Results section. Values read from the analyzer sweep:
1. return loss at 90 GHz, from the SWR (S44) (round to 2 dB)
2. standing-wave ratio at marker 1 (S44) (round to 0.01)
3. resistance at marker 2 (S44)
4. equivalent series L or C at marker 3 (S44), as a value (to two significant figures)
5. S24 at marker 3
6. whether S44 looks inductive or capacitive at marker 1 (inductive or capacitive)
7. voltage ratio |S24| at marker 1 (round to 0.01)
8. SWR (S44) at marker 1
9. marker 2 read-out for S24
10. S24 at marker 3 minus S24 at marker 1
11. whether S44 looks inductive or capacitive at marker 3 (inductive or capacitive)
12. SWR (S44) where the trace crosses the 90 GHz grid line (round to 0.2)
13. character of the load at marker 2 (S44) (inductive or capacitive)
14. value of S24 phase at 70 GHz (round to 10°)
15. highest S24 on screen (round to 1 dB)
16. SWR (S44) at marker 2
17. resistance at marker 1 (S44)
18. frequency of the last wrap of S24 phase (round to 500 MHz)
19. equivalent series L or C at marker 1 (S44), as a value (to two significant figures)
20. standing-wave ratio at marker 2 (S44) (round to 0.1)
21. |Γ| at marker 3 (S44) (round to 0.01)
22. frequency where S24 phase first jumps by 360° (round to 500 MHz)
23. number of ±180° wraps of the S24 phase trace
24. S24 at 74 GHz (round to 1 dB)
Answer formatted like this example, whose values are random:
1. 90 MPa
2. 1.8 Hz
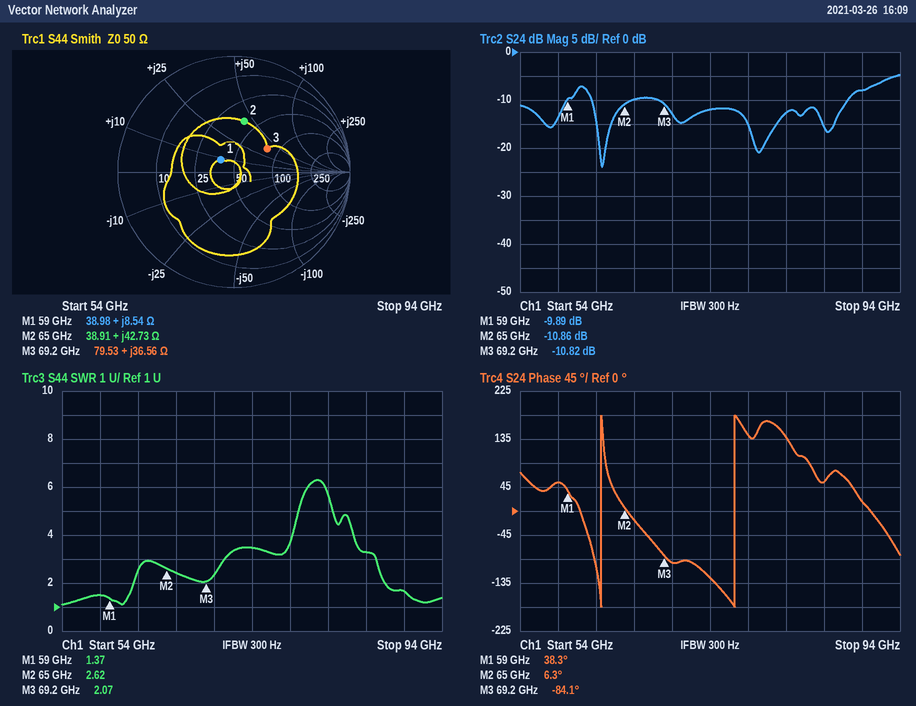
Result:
1. 12 dB
2. 1.37
3. 38.91 Ω
4. 84 pH
5. -10.82 dB
6. inductive
7. 0.32
8. 1.37
9. -10.86 dB
10. -0.93 dB
11. inductive
12. 1.6
13. inductive
14. -100°
15. -5 dB
16. 2.62
17. 38.98 Ω
18. 76.5 GHz
19. 23 pH
20. 2.6
21. 0.35
22. 62.5 GHz
23. 2
24. -12 dB
